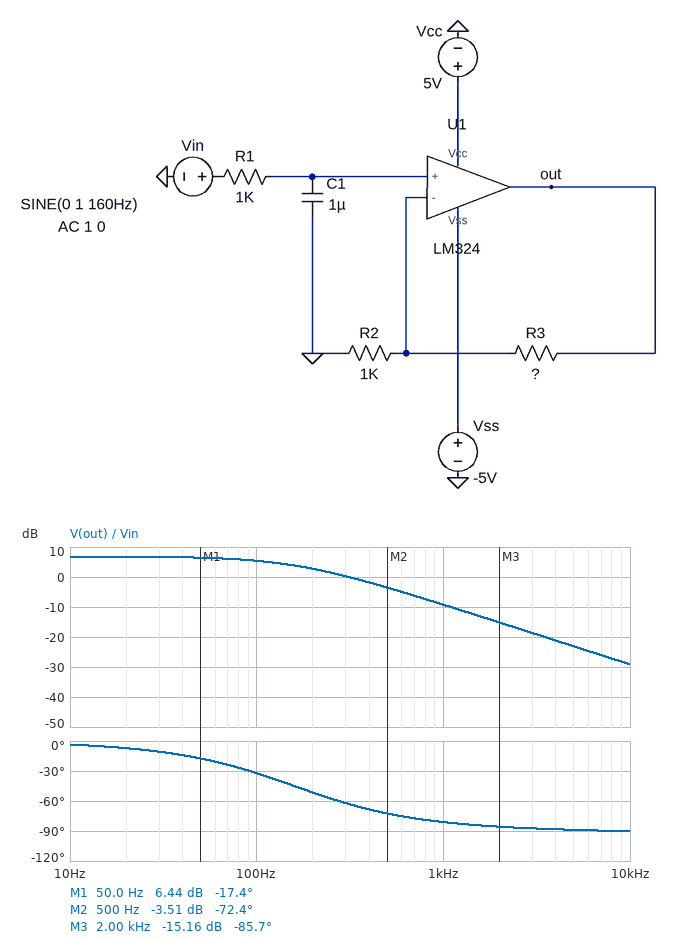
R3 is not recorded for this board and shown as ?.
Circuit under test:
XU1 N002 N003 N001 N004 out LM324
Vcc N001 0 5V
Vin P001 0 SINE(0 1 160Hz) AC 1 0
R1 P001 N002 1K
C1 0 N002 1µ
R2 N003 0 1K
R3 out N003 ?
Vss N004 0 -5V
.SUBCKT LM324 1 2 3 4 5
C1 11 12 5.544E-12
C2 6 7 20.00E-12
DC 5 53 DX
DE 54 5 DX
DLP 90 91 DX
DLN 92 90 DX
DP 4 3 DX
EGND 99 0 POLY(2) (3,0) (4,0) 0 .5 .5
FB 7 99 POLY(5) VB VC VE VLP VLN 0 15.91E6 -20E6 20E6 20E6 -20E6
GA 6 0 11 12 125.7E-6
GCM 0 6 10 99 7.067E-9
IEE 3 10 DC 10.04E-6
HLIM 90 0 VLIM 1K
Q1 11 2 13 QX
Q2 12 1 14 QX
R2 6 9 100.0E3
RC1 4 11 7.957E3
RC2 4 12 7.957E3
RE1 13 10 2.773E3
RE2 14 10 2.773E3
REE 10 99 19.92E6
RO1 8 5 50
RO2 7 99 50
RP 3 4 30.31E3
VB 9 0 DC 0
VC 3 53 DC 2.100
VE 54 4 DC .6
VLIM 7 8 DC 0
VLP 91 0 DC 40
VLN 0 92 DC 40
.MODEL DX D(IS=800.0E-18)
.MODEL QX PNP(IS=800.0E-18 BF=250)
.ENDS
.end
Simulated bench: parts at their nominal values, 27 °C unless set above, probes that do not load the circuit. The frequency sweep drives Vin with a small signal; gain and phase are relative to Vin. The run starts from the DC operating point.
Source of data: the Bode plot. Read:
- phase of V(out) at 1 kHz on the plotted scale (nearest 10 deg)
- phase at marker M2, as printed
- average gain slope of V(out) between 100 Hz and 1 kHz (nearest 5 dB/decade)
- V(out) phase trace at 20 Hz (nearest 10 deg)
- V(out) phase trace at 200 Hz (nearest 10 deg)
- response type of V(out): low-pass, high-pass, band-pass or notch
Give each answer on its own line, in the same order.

-80 deg
-72.4 deg
-15 dB/decade
-10 deg
-50 deg
low-pass
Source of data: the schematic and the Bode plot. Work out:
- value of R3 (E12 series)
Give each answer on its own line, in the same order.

1.2 kΩ
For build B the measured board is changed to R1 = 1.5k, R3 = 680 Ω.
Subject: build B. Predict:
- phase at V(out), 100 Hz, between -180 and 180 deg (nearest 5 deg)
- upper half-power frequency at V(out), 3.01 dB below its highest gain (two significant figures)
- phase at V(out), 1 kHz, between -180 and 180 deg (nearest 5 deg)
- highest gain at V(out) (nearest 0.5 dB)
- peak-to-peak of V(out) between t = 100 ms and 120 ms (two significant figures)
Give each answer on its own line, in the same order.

-45 deg
110 Hz
-85 deg
4.5 dB
1.9 V
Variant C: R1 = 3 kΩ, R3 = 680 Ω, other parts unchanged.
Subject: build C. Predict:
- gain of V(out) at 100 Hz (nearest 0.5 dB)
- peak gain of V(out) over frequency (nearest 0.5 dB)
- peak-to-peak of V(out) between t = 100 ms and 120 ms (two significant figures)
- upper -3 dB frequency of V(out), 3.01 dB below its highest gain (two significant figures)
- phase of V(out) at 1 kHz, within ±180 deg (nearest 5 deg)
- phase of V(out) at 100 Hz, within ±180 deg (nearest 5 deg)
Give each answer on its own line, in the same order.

-2.0 dB
4.5 dB
1.1 V
53 Hz
-85 deg
-60 deg
